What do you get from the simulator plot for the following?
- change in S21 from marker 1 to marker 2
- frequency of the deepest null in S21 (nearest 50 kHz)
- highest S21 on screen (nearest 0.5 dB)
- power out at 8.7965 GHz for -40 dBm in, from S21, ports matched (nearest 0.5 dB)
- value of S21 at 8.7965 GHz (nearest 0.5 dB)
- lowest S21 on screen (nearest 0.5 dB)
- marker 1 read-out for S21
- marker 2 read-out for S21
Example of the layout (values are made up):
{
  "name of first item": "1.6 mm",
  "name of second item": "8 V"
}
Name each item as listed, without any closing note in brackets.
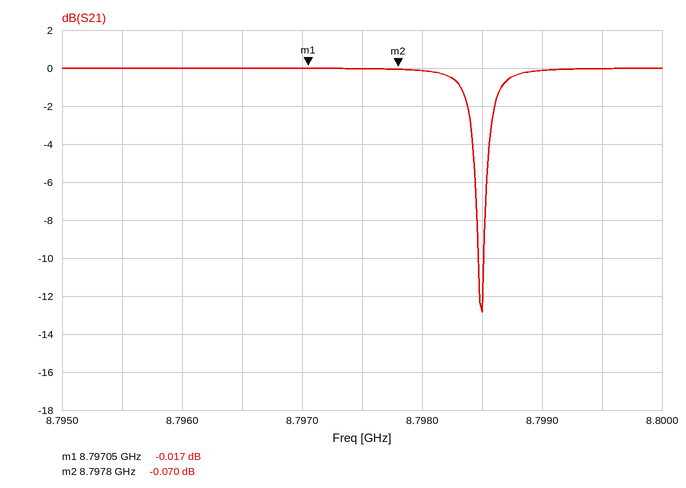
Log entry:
{
  "change in S21 from marker 1 to marker 2": "-0.053 dB",
  "frequency of the deepest null in S21": "8.79850 GHz",
  "highest S21 on screen": "0.0 dB",
  "power out at 8.7965 GHz for -40 dBm in, from S21, ports matched": "-40.0 dBm",
  "value of S21 at 8.7965 GHz": "0.0 dB",
  "lowest S21 on screen": "-13.0 dB",
  "marker 1 read-out for S21": "-0.017 dB",
  "marker 2 read-out for S21": "-0.070 dB"
}
